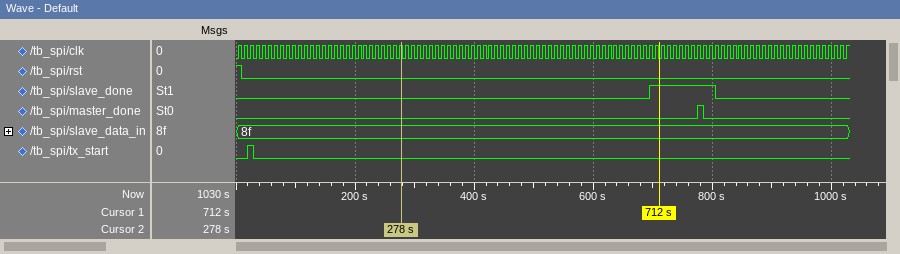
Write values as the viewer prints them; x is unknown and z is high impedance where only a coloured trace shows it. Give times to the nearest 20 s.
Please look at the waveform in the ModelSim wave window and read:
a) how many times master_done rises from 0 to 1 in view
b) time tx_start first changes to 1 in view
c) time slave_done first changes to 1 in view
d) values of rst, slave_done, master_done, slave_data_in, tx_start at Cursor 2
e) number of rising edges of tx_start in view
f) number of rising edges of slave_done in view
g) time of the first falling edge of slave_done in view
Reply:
1
20 s
700 s
rst=0, slave_done=0, master_done=0, slave_data_in=8f, tx_start=0
1
1
800 s
